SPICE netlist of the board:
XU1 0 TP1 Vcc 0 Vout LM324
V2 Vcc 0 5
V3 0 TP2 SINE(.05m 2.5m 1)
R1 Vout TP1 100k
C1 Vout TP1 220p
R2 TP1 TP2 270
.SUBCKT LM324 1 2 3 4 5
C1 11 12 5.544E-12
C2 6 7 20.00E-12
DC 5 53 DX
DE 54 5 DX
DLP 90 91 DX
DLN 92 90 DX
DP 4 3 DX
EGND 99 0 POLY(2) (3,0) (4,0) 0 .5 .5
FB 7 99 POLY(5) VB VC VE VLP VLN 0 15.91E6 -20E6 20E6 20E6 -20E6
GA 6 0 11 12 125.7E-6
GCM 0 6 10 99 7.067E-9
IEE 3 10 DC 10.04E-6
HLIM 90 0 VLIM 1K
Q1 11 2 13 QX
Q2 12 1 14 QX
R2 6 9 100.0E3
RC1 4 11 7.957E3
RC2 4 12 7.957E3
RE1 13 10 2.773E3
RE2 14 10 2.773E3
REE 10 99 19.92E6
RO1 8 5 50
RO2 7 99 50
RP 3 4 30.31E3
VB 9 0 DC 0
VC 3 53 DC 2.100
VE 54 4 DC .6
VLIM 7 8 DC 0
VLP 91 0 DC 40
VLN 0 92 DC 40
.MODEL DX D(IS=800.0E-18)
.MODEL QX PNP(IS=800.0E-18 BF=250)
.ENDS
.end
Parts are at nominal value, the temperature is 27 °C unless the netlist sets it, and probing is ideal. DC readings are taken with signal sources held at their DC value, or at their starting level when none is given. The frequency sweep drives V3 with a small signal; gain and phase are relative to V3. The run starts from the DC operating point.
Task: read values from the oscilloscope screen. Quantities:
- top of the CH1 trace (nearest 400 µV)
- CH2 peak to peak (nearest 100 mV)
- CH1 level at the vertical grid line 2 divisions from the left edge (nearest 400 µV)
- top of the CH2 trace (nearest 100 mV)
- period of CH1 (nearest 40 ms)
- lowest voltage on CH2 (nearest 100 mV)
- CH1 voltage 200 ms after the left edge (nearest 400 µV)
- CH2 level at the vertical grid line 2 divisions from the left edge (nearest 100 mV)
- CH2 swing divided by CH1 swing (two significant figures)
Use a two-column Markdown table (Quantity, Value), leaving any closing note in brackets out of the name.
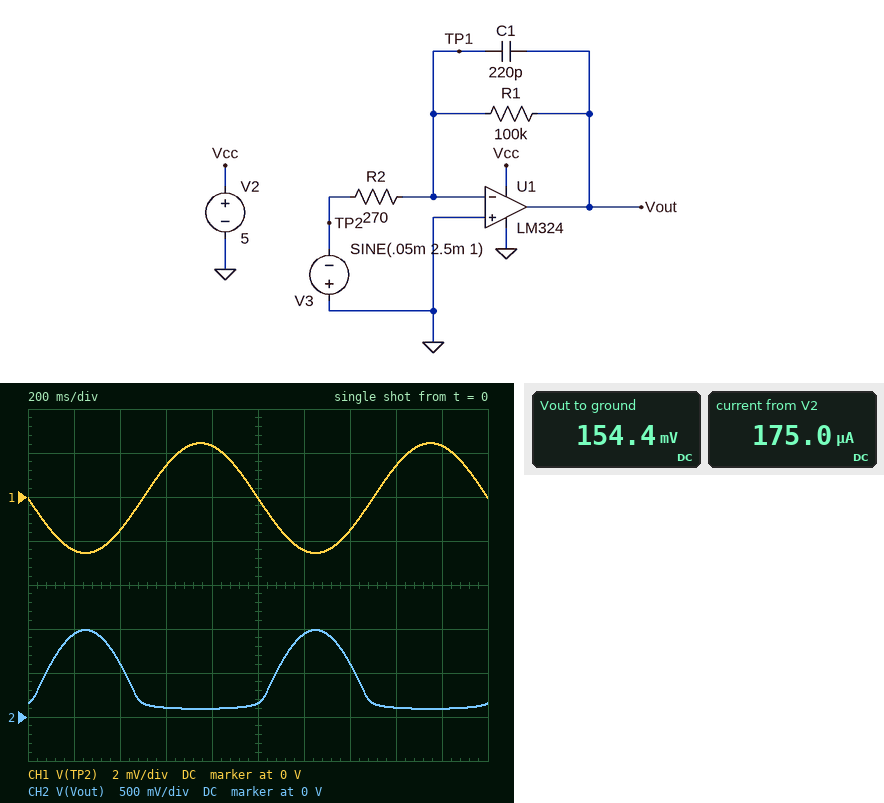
| Quantity | Value |
|---|---|
| top of the CH1 trace | 2.4 mV |
| CH2 peak to peak | 900 mV |
| CH1 level at the vertical grid line 2 divisions from the left edge | -1.6 mV |
| top of the CH2 trace | 1.0 V |
| period of CH1 | 1.00 s |
| lowest voltage on CH2 | 100 mV |
| CH1 voltage 200 ms after the left edge | -2.4 mV |
| CH2 level at the vertical grid line 2 divisions from the left edge | 600 mV |
| CH2 swing divided by CH1 swing | 180 |
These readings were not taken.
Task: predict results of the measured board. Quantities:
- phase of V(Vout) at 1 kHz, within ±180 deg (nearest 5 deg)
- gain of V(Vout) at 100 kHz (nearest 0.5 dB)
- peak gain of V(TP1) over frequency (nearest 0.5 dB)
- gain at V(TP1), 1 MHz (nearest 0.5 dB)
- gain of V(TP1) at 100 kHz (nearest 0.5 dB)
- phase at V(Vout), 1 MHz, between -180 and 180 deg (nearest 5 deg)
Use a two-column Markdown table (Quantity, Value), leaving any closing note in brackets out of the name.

| Quantity | Value |
|---|---|
| phase of V(Vout) at 1 kHz, within ±180 deg | -5 deg |
| gain of V(Vout) at 100 kHz | 16.5 dB |
| peak gain of V(TP1) over frequency | -2.0 dB |
| gain at V(TP1), 1 MHz | -2.0 dB |
| gain of V(TP1) at 100 kHz | -2.5 dB |
| phase at V(Vout), 1 MHz, between -180 and 180 deg | -130 deg |
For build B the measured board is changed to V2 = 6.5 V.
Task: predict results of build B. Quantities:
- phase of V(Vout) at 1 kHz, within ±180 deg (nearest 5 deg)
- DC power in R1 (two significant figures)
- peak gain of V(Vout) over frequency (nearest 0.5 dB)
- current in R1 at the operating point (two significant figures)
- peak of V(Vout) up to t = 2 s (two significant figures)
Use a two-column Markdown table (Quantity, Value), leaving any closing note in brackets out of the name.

| Quantity | Value |
|---|---|
| phase of V(Vout) at 1 kHz, within ±180 deg | -10 deg |
| DC power in R1 | 250 nW |
| peak gain of V(Vout) over frequency | 39.5 dB |
| current in R1 at the operating point | 1.6 µA |
| peak of V(Vout) up to t = 2 s | 1.0 V |
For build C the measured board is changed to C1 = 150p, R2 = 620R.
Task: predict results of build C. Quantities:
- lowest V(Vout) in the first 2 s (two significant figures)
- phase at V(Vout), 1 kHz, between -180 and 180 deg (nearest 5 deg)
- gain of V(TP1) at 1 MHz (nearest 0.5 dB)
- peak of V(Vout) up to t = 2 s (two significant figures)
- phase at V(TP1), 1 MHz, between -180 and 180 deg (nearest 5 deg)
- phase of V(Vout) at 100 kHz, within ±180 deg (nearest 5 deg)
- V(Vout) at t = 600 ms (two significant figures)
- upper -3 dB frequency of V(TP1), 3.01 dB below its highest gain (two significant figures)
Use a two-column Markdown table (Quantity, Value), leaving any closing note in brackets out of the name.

| Quantity | Value |
|---|---|
| lowest V(Vout) in the first 2 s | 90 mV |
| phase at V(Vout), 1 kHz, between -180 and 180 deg | -5 deg |
| gain of V(TP1) at 1 MHz | -3.0 dB |
| peak of V(Vout) up to t = 2 s | 430 mV |
| phase at V(TP1), 1 MHz, between -180 and 180 deg | 165 deg |
| phase of V(Vout) at 100 kHz, within ±180 deg | -85 deg |
| V(Vout) at t = 600 ms | 100 mV |
| upper -3 dB frequency of V(TP1), 3.01 dB below its highest gain | 2.5 MHz |
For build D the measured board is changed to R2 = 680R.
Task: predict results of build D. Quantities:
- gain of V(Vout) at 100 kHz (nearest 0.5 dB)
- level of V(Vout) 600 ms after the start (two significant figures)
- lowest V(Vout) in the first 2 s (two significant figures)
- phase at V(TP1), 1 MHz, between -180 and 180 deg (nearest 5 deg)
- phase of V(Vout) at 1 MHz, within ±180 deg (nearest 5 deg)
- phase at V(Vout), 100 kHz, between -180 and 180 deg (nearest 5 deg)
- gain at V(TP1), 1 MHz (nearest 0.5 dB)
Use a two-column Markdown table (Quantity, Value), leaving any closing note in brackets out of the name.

| Quantity | Value |
|---|---|
| gain of V(Vout) at 100 kHz | 12.5 dB |
| level of V(Vout) 600 ms after the start | 100 mV |
| lowest V(Vout) in the first 2 s | 90 mV |
| phase at V(TP1), 1 MHz, between -180 and 180 deg | 160 deg |
| phase of V(Vout) at 1 MHz, within ±180 deg | -140 deg |
| phase at V(Vout), 100 kHz, between -180 and 180 deg | -85 deg |
| gain at V(TP1), 1 MHz | -4.5 dB |
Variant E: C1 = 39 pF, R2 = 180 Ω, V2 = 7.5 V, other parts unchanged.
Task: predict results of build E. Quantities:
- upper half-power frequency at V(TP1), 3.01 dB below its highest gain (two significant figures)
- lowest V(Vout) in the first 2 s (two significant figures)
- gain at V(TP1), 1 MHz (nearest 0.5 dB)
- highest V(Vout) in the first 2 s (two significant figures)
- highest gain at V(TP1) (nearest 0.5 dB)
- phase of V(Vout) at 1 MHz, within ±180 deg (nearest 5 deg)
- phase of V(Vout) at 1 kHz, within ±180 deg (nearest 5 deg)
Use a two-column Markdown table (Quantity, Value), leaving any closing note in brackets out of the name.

| Quantity | Value |
|---|---|
| upper half-power frequency at V(TP1), 3.01 dB below its highest gain | 20 MHz |
| lowest V(Vout) in the first 2 s | 95 mV |
| gain at V(TP1), 1 MHz | -0.5 dB |
| highest V(Vout) in the first 2 s | 1.5 V |
| highest gain at V(TP1) | 0 dB |
| phase of V(Vout) at 1 MHz, within ±180 deg | -120 deg |
| phase of V(Vout) at 1 kHz, within ±180 deg | -15 deg |
